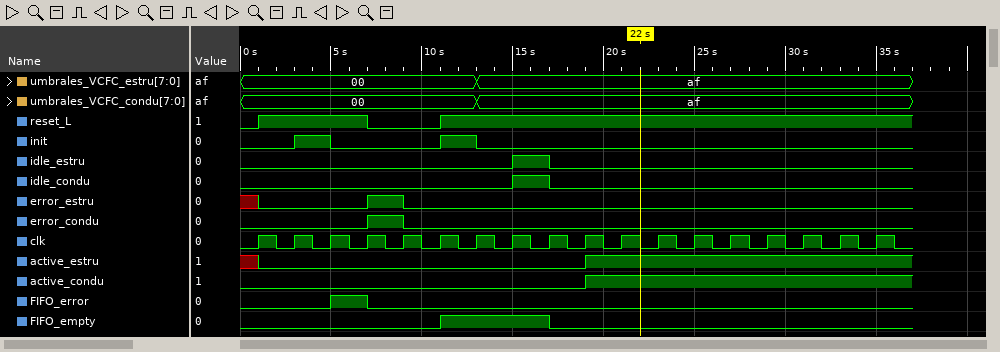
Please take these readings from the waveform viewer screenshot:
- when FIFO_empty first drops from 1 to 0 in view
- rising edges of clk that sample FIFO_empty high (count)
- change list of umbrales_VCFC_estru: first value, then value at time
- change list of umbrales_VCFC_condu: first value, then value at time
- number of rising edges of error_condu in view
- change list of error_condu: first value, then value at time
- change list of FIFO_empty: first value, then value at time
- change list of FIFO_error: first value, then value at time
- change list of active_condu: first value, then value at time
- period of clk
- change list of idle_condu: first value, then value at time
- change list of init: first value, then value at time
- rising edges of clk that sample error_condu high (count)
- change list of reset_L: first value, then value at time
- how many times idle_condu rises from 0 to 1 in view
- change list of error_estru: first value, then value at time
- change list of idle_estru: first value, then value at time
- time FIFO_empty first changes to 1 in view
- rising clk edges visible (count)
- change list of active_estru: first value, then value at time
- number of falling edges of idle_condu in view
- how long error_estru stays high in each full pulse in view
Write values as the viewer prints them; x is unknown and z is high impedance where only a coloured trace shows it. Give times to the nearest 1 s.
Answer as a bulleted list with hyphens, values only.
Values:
- 17 s
- 3
- 00, af at 13 s
- 00, af at 13 s
- 1
- 0, 1 at 7 s, 0 at 9 s
- 0, 1 at 11 s, 0 at 17 s
- 0, 1 at 5 s, 0 at 7 s
- 0, 1 at 19 s
- 2 s
- 0, 1 at 15 s, 0 at 17 s
- 0, 1 at 3 s, 0 at 5 s, 1 at 11 s, 0 at 13 s
- 1
- 0, 1 at 1 s, 0 at 7 s, 1 at 11 s
- 1
- x, 0 at 1 s, 1 at 7 s, 0 at 9 s
- 0, 1 at 15 s, 0 at 17 s
- 11 s
- 18
- x, 0 at 1 s, 1 at 19 s
- 1
- 2 s
